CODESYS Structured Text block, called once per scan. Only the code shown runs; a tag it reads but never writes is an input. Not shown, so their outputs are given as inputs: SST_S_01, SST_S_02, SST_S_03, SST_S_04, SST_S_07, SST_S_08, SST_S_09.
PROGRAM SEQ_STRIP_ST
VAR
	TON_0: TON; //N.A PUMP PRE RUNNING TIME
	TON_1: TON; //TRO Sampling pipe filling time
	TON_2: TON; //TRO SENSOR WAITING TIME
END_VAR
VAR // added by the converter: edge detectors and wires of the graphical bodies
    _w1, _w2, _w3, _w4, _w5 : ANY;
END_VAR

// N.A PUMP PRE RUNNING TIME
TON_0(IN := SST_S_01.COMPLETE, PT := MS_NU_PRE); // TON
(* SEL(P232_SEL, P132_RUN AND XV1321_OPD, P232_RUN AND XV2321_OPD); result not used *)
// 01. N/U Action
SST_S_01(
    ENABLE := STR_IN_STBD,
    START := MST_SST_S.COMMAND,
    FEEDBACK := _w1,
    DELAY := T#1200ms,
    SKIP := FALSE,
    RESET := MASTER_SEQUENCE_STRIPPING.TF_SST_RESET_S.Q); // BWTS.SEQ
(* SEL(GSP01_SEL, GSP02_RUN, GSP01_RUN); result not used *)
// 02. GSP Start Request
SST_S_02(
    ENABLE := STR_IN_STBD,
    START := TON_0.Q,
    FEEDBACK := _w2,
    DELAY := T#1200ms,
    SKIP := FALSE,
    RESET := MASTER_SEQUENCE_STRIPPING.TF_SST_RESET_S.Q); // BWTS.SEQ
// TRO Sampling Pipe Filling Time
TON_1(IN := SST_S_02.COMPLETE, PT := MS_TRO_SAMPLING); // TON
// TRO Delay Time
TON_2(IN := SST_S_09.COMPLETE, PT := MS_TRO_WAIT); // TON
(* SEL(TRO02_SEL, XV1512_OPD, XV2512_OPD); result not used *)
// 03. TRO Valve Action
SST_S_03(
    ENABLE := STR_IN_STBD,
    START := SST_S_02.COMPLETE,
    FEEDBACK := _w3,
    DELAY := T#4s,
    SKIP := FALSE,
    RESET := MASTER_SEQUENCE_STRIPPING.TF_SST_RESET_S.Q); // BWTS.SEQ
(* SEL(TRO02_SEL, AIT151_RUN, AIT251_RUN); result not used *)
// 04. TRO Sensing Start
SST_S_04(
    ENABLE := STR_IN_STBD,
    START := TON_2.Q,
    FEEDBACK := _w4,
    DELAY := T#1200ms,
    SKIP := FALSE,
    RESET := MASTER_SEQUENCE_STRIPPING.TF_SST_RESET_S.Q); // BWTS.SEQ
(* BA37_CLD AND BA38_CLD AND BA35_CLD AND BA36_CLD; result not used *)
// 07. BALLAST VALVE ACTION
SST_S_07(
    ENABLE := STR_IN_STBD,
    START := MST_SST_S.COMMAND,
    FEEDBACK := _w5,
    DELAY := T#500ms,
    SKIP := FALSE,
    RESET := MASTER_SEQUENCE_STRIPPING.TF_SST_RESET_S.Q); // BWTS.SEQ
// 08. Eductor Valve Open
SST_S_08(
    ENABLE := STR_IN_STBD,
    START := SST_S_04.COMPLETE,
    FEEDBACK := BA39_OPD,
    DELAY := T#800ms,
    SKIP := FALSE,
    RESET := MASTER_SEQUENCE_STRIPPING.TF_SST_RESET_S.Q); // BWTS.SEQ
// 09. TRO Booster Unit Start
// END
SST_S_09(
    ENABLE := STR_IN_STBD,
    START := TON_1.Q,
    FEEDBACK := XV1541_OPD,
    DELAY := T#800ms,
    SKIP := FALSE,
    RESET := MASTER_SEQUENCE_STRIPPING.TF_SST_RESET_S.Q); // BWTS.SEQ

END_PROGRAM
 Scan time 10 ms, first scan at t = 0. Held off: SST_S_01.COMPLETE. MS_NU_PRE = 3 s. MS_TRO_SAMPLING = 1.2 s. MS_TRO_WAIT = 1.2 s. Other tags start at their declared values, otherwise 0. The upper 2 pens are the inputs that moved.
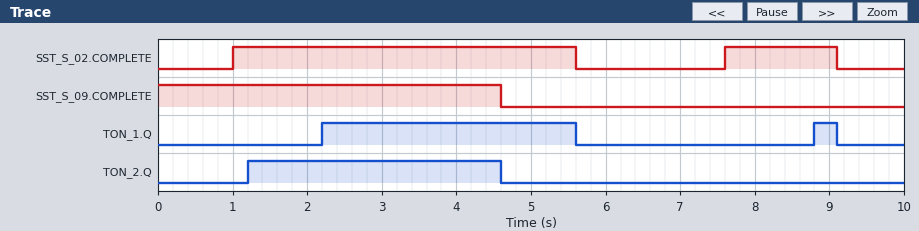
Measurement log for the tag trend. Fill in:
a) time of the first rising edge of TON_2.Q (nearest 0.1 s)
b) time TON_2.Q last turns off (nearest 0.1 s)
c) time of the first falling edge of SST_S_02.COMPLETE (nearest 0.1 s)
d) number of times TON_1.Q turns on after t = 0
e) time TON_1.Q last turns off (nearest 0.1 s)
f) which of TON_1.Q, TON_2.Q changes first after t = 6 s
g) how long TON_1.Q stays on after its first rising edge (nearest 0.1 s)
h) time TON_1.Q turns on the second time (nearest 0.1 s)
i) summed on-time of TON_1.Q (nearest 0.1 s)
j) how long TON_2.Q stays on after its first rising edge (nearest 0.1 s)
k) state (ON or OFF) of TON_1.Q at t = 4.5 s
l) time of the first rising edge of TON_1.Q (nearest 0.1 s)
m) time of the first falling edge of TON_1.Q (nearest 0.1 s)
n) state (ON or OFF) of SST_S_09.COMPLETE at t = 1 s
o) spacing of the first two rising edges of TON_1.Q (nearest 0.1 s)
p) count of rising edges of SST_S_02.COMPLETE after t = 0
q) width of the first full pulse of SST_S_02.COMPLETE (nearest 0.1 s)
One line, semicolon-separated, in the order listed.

1.2 s; 4.6 s; 5.6 s; 2; 9.1 s; TON_1.Q; 3.4 s; 8.8 s; 3.7 s; 3.4 s; ON; 2.2 s; 5.6 s; ON; 6.6 s; 2; 4.6 s
